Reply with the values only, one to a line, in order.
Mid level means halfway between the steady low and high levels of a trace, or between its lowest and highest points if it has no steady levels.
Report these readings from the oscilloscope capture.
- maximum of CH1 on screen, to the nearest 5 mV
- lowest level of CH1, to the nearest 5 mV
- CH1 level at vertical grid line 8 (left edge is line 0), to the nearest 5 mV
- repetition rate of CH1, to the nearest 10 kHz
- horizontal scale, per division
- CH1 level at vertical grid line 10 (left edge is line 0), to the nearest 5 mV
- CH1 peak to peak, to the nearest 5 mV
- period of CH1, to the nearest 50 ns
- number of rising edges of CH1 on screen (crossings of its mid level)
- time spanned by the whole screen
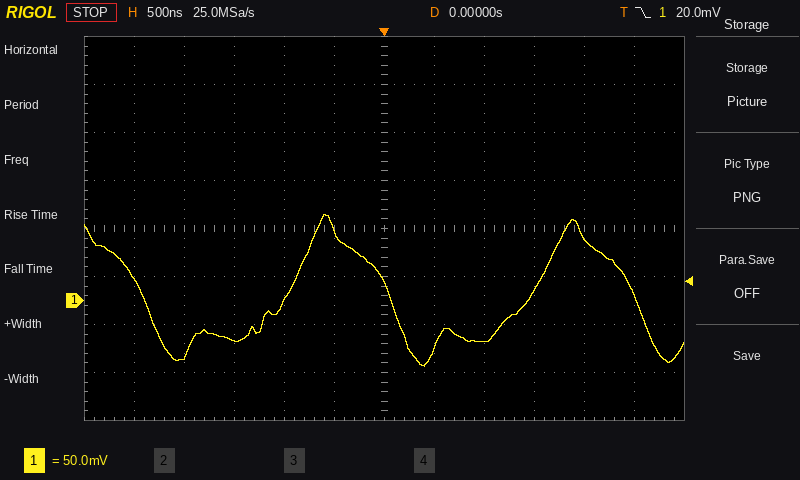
90 mV
-70 mV
-45 mV
410 kHz
500 ns
65 mV
160 mV
2.45 µs
2
6 µs
